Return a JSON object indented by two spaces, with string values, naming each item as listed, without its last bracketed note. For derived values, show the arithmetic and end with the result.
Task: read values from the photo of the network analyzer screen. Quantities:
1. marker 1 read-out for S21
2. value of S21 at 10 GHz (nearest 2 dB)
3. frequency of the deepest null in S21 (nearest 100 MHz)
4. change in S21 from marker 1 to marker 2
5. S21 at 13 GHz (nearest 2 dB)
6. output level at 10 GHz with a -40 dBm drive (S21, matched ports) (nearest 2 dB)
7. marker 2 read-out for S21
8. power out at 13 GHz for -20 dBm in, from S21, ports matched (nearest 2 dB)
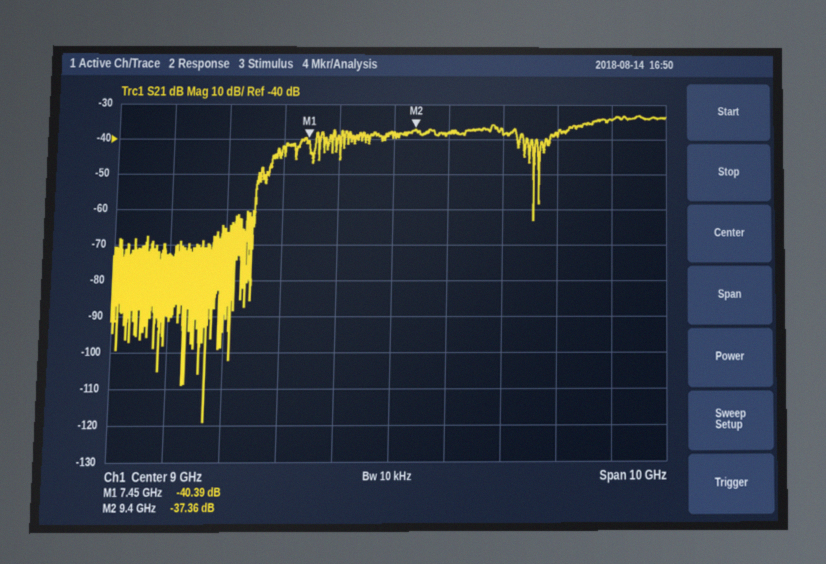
{
  "marker 1 read-out for S21": "-40.39 dB",
  "value of S21 at 10 GHz": "-38 dB",
  "frequency of the deepest null in S21": "5.7 GHz",
  "change in S21 from marker 1 to marker 2": "-37.36 − (-40.39) = 3.03 dB",
  "S21 at 13 GHz": "-34 dB",
  "output level at 10 GHz with a -40 dBm drive (S21, matched ports)": "-40 dBm + (-38 dB) = -78 dBm",
  "marker 2 read-out for S21": "-37.36 dB",
  "power out at 13 GHz for -20 dBm in, from S21, ports matched": "-20 dBm + (-34 dB) = -54 dBm"
}
